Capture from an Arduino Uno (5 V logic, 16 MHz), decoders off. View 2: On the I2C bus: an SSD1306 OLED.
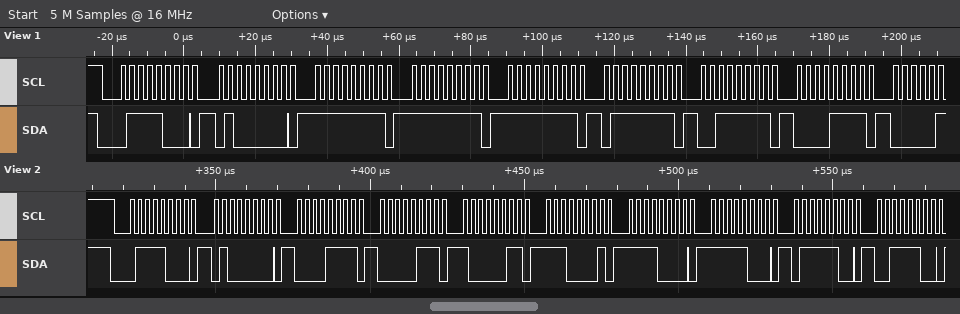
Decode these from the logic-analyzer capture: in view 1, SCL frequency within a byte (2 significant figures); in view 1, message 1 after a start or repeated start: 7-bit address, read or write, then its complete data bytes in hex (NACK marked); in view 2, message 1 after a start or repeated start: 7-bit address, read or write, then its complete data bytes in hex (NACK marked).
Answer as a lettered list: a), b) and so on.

a) 400 kHz
b) 0x3C write: 40 FF FF FF 7F 3F 0F
c) 0x3C write: 40 0F 07 83 E1 F0 F8 7C 3C
